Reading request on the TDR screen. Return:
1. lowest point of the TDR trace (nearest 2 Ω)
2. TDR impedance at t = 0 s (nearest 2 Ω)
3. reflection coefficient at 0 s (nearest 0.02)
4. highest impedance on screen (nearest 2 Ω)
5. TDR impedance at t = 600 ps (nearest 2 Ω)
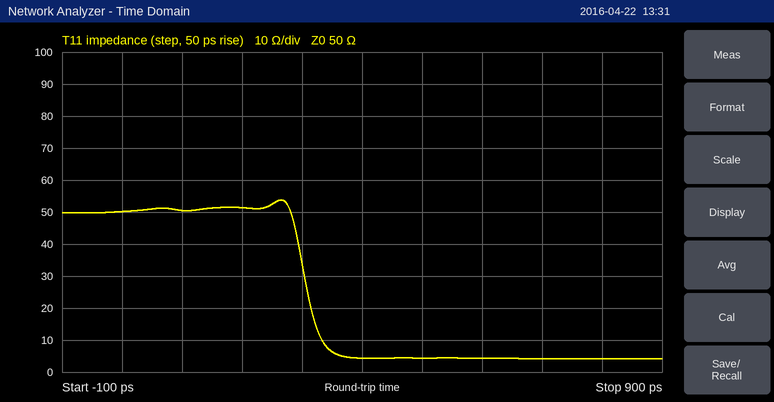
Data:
4 Ω
50 Ω
0.00
54 Ω
4 Ω
